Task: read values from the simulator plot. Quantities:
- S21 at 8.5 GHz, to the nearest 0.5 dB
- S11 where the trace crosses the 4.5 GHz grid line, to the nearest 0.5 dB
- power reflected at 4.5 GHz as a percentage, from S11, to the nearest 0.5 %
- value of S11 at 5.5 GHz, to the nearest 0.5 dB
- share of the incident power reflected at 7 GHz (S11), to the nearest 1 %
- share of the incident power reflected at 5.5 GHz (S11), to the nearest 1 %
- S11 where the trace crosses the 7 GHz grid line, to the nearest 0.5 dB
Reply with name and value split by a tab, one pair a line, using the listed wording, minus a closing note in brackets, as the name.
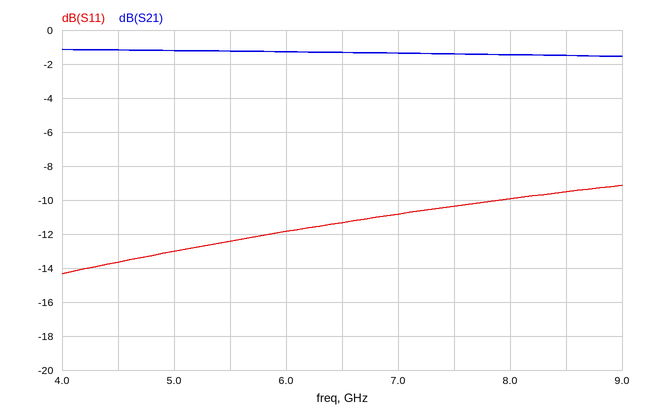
S21 at 8.5 GHz, to the nearest 0.5 dB	-1.5 dB
S11 where the trace crosses the 4.5 GHz grid line, to the nearest 0.5 dB	-13.5 dB
power reflected at 4.5 GHz as a percentage, from S11, to the nearest 0.5 %	4.5 %
value of S11 at 5.5 GHz, to the nearest 0.5 dB	-12.5 dB
share of the incident power reflected at 7 GHz (S11), to the nearest 1 %	8 %
share of the incident power reflected at 5.5 GHz (S11), to the nearest 1 %	6 %
S11 where the trace crosses the 7 GHz grid line, to the nearest 0.5 dB	-11.0 dB
